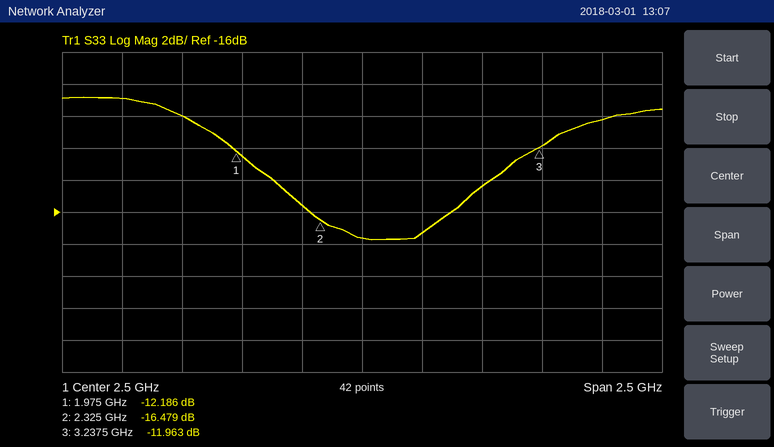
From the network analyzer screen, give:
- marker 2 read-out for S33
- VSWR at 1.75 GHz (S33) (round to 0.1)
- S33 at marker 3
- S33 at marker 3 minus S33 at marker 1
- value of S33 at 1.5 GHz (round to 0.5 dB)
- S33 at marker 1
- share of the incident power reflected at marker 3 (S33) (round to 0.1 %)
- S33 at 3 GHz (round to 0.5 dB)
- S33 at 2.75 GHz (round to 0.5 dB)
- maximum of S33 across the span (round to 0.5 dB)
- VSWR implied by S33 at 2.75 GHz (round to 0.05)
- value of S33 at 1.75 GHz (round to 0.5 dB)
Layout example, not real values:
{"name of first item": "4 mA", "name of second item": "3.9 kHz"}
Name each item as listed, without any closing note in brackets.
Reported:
{"marker 2 read-out for S33": "-16.479 dB", "VSWR at 1.75 GHz (S33)": "1.9", "S33 at marker 3": "-11.963 dB", "S33 at marker 3 minus S33 at marker 1": "0.223 dB", "value of S33 at 1.5 GHz": "-9.0 dB", "S33 at marker 1": "-12.186 dB", "share of the incident power reflected at marker 3 (S33)": "6.4 %", "S33 at 3 GHz": "-14.5 dB", "S33 at 2.75 GHz": "-17.5 dB", "maximum of S33 across the span": "-9.0 dB", "VSWR implied by S33 at 2.75 GHz": "1.30", "value of S33 at 1.75 GHz": "-10.0 dB"}
